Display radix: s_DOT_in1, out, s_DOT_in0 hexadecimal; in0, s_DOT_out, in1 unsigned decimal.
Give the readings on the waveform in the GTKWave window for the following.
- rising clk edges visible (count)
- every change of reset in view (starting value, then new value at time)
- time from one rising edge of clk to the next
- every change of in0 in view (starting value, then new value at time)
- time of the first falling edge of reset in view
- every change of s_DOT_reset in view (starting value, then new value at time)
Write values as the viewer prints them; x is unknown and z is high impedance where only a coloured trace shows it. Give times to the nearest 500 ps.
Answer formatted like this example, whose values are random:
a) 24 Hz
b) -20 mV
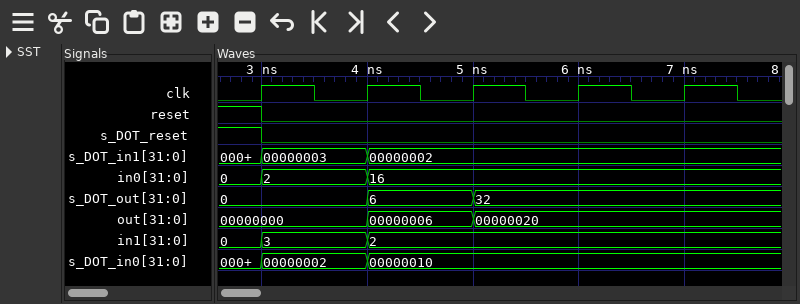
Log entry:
a) 5
b) 1, 0 at 3000 ps
c) 1000 ps
d) 0, 2 at 3000 ps, 16 at 4000 ps
e) 3000 ps
f) 1, 0 at 3000 ps
